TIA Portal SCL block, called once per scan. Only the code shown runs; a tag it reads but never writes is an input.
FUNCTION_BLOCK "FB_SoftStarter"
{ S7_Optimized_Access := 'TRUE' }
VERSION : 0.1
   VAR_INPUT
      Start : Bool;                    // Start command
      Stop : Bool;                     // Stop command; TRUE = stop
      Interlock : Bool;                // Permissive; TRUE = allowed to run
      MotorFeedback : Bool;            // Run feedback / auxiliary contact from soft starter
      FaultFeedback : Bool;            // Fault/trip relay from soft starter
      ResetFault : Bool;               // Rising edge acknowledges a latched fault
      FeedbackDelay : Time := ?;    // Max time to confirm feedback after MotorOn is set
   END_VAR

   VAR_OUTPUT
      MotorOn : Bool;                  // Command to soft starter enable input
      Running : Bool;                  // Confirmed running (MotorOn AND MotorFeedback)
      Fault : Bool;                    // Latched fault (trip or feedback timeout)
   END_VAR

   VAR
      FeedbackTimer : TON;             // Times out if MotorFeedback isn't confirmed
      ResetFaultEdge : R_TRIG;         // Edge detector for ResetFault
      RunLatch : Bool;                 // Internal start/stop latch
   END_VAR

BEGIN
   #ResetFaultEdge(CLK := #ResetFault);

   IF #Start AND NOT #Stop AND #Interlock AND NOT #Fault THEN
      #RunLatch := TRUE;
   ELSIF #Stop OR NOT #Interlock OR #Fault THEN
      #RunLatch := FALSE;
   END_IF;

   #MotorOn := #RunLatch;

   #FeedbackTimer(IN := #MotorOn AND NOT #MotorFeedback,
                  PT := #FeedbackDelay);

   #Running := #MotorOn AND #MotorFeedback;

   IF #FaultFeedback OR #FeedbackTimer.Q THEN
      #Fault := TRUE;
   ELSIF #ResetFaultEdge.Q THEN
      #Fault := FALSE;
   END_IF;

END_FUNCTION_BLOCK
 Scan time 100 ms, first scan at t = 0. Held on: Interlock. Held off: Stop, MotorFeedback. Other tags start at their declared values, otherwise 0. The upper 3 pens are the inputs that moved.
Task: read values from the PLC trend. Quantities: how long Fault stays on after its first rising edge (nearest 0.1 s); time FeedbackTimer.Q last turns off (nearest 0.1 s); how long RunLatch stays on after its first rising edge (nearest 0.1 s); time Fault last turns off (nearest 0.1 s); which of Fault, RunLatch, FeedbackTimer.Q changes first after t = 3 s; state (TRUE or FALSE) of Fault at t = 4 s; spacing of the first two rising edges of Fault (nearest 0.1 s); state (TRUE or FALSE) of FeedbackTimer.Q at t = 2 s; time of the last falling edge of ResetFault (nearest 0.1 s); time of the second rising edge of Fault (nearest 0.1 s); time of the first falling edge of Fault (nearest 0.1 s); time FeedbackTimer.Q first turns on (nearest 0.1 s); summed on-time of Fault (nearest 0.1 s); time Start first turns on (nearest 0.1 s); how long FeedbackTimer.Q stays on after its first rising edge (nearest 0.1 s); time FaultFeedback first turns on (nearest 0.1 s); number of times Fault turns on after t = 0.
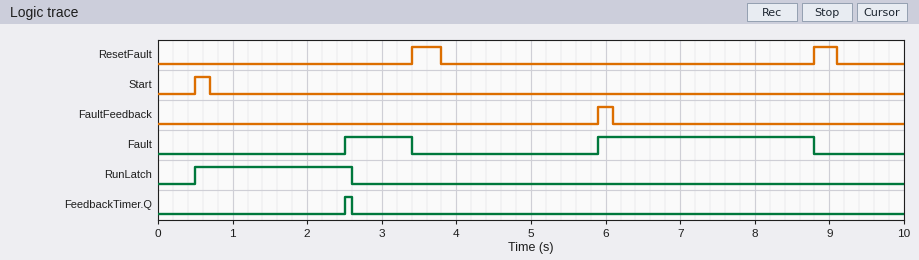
0.9 s
2.6 s
2.1 s
8.8 s
Fault
FALSE
3.4 s
FALSE
9.1 s
5.9 s
3.4 s
2.5 s
3.8 s
0.5 s
0.1 s
5.9 s
2
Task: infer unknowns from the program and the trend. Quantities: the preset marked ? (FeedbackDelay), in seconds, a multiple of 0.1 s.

2.0 s
